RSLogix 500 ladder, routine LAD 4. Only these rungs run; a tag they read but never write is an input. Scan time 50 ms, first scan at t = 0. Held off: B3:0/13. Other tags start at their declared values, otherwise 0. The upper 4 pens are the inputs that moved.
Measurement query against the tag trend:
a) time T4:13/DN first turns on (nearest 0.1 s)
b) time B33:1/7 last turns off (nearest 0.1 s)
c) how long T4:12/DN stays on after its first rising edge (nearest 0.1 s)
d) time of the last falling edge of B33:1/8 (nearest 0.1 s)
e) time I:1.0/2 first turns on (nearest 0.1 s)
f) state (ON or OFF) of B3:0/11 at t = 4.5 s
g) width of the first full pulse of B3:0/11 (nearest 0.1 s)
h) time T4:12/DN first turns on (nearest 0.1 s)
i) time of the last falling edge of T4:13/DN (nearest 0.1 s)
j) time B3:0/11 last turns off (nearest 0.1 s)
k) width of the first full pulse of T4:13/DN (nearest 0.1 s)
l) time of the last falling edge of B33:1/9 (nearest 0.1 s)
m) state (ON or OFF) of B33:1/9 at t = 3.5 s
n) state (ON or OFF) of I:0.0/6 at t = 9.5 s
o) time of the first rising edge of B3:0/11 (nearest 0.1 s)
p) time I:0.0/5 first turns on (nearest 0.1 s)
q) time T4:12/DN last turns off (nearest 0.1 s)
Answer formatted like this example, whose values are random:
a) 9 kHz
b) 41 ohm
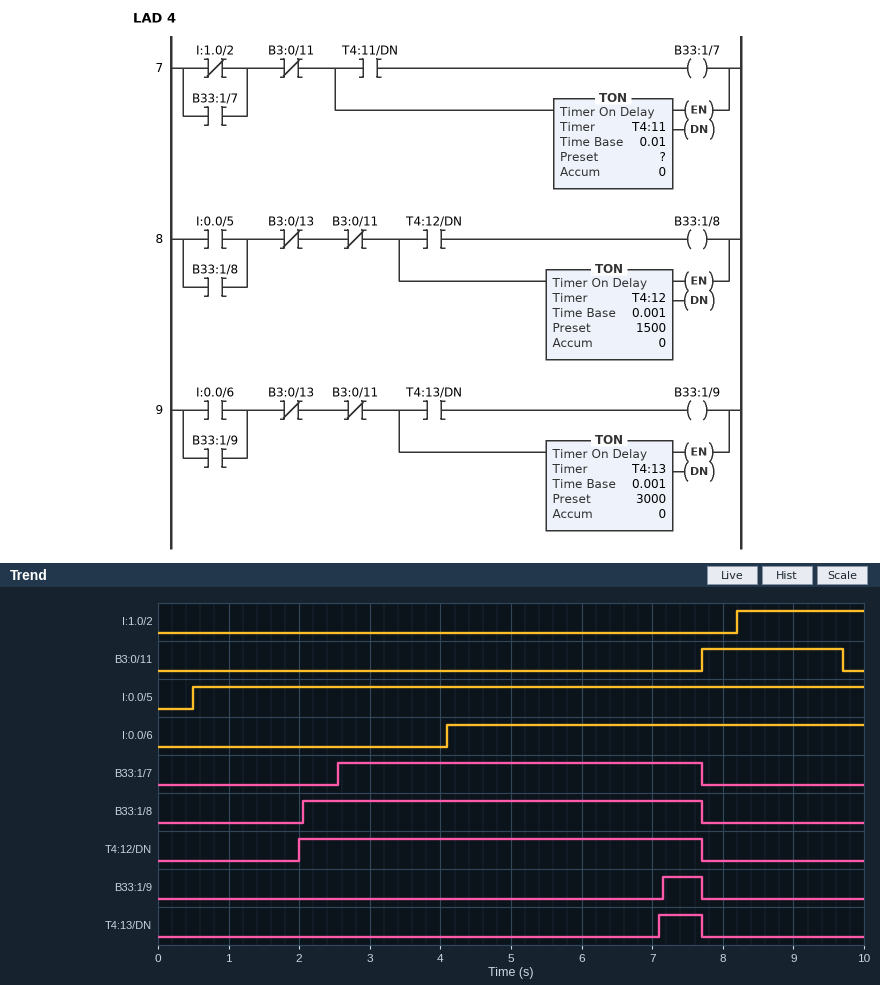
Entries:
a) 7.1 s
b) 7.7 s
c) 5.7 s
d) 7.7 s
e) 8.2 s
f) OFF
g) 2.0 s
h) 2.0 s
i) 7.7 s
j) 9.7 s
k) 0.6 s
l) 7.7 s
m) OFF
n) ON
o) 7.7 s
p) 0.5 s
q) 7.7 s
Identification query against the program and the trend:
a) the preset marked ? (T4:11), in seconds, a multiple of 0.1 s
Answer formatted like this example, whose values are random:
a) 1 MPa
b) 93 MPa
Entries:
a) 2.5 s
